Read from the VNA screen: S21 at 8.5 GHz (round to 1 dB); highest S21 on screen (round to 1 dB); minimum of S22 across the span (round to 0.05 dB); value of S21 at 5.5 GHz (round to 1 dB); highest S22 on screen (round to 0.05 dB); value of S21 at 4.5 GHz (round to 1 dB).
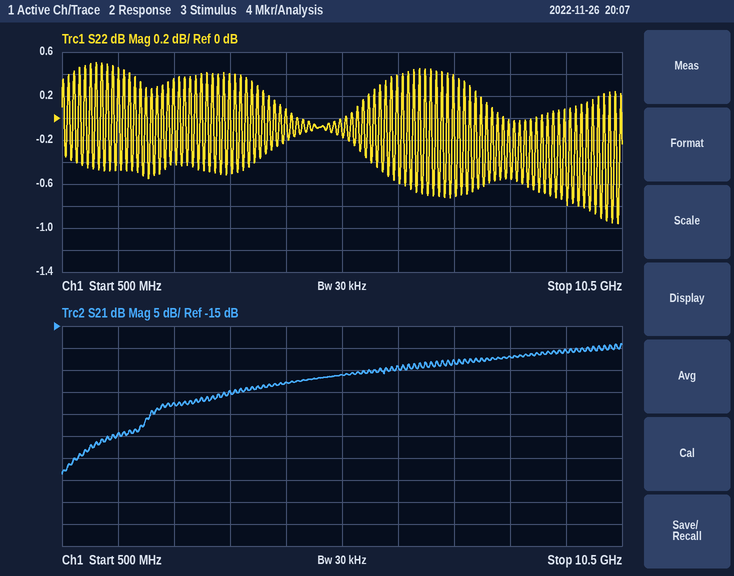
-22 dB
-19 dB
-0.95 dB
-26 dB
0.50 dB
-28 dB
